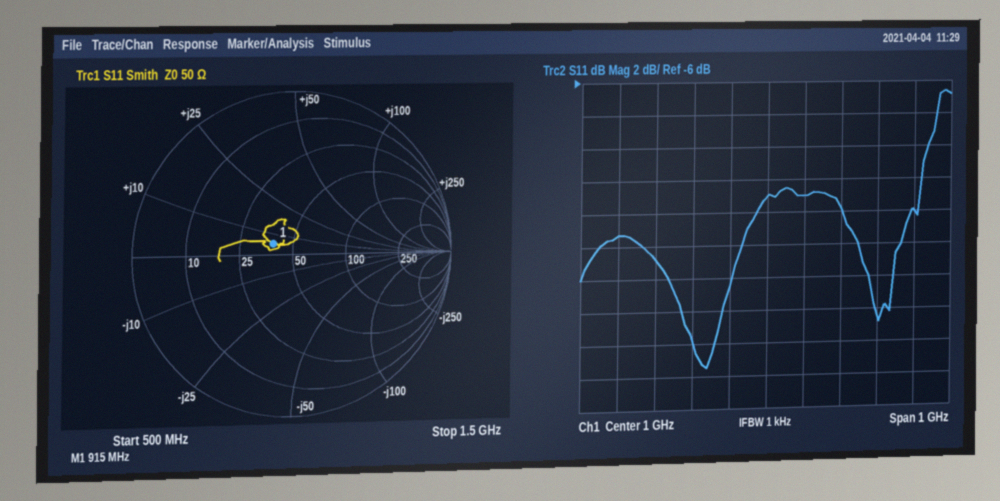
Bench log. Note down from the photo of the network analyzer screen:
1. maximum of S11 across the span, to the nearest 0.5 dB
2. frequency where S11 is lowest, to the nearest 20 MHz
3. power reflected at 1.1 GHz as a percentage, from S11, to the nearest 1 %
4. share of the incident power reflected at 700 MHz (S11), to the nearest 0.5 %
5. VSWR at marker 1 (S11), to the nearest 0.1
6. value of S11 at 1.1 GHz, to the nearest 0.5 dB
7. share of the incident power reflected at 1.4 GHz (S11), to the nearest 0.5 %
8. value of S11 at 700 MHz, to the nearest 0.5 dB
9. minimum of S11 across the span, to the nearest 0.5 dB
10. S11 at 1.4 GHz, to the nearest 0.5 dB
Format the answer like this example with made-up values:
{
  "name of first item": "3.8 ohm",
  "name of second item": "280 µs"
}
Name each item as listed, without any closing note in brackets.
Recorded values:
{
  "maximum of S11 across the span, to the nearest 0.5 dB": "-6.5 dB",
  "frequency where S11 is lowest, to the nearest 20 MHz": "840 MHz",
  "power reflected at 1.1 GHz as a percentage, from S11, to the nearest 1 %": "5 %",
  "share of the incident power reflected at 700 MHz (S11), to the nearest 0.5 %": "2.0 %",
  "VSWR at marker 1 (S11), to the nearest 0.1": "1.3",
  "value of S11 at 1.1 GHz, to the nearest 0.5 dB": "-13.0 dB",
  "share of the incident power reflected at 1.4 GHz (S11), to the nearest 0.5 %": "4.0 %",
  "value of S11 at 700 MHz, to the nearest 0.5 dB": "-17.0 dB",
  "minimum of S11 across the span, to the nearest 0.5 dB": "-23.5 dB",
  "S11 at 1.4 GHz, to the nearest 0.5 dB": "-14.0 dB"
}
